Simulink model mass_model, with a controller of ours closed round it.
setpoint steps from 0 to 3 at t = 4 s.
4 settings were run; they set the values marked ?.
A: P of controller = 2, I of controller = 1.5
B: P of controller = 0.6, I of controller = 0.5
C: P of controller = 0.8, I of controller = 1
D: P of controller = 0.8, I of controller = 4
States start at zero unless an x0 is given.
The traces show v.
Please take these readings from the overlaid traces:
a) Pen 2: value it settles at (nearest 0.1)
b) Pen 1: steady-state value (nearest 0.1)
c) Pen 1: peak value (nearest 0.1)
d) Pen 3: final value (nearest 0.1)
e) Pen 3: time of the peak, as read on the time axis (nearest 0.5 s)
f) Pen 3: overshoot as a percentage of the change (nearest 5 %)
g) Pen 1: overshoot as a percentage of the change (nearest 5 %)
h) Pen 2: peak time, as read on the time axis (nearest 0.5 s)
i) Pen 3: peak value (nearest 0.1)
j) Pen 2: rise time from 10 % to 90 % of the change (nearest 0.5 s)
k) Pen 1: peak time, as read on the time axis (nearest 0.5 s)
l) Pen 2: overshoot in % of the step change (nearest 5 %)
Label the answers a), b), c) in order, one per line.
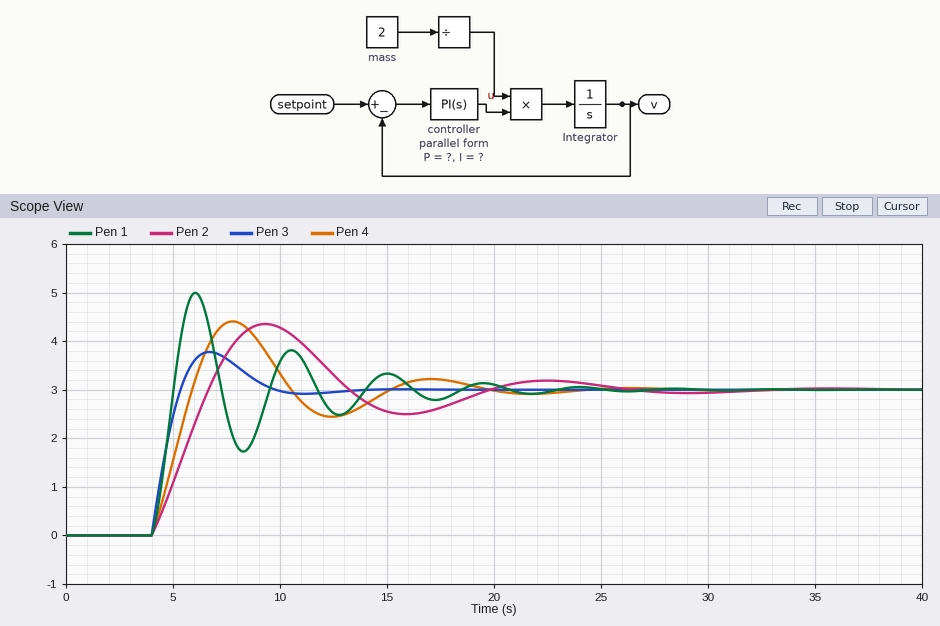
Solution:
a) 3.0
b) 3.0
c) 5.0
d) 3.0
e) 6.5 s
f) 25 %
g) 65 %
h) 9.5 s
i) 3.8
j) 2.0 s
k) 6.0 s
l) 45 %
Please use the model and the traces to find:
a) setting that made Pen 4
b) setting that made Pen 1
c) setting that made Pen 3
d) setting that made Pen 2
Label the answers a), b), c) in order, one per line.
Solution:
a) C
b) D
c) A
d) B
